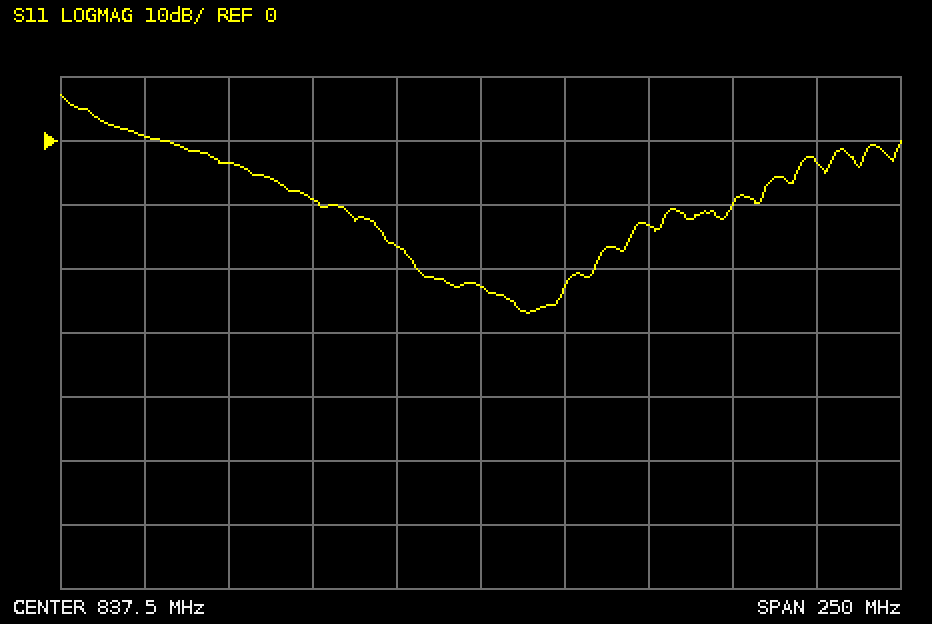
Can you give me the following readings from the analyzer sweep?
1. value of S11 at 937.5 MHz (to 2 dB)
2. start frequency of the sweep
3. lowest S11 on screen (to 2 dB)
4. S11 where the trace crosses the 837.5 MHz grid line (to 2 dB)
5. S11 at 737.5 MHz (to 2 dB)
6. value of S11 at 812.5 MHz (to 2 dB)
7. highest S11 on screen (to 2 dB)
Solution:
-4 dB
712.5 MHz
-26 dB
-22 dB
0 dB
-16 dB
8 dB
